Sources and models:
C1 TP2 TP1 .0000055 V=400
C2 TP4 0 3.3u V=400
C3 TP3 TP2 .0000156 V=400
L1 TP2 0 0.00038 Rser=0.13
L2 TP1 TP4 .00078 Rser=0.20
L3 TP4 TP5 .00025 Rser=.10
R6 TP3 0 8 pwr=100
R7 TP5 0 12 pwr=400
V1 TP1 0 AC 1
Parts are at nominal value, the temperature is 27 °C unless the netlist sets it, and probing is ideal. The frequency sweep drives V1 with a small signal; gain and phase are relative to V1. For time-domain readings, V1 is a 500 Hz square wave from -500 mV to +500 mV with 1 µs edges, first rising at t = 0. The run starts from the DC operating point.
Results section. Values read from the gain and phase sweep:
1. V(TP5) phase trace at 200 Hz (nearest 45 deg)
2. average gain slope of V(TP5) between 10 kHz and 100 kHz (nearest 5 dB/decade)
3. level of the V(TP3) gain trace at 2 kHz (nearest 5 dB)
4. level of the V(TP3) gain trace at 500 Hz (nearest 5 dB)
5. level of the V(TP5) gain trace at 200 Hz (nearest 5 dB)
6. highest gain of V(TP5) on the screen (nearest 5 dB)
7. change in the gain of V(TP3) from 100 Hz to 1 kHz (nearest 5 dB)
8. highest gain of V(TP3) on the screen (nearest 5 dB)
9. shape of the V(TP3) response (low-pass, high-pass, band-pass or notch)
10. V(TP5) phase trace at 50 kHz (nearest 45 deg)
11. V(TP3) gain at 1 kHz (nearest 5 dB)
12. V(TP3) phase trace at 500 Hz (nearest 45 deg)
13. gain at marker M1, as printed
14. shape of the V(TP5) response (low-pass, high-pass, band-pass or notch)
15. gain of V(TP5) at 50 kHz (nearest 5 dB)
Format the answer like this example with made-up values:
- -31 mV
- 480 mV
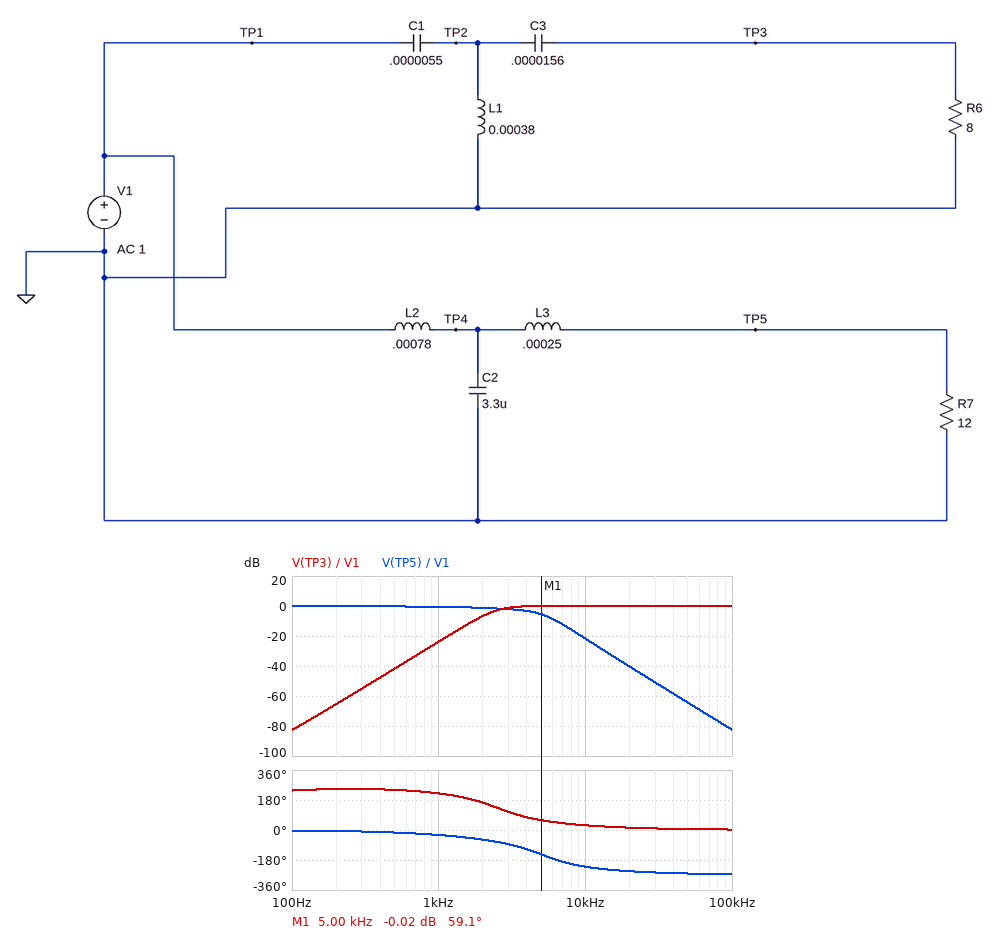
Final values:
- 0 deg
- -60 dB/decade
- -5 dB
- -40 dB
- 0 dB
- 0 dB
- 60 dB
- 0 dB
- high-pass
- -270 deg
- -25 dB
- 225 deg
- -0.02 dB
- low-pass
- -65 dB
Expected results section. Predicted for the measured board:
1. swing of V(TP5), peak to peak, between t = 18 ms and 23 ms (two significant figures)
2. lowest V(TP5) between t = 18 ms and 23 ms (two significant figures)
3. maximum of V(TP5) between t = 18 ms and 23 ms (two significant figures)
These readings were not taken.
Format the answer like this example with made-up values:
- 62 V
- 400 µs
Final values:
- 980 mV
- -490 mV
- 490 mV
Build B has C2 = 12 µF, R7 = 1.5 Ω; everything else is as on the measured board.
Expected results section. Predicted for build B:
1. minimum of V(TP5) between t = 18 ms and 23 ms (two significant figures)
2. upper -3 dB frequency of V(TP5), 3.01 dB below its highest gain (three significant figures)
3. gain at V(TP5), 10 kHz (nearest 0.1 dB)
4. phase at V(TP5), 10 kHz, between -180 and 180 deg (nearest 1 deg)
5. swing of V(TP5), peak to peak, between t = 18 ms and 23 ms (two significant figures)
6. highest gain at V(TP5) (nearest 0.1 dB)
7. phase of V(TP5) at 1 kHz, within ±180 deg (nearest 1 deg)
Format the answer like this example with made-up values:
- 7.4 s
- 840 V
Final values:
- -290 mV
- 287 Hz
- -50.8 dB
- 97 deg
- 590 mV
- -1.6 dB
- -79 deg
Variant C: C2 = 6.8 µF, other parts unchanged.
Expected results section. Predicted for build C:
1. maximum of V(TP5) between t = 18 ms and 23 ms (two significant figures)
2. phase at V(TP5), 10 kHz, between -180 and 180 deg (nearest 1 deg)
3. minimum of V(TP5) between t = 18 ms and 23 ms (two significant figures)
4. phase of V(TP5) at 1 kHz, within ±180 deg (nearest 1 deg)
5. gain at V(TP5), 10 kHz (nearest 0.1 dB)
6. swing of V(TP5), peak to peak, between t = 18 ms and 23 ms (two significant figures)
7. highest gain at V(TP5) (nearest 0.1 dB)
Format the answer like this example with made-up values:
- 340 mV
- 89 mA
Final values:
- 650 mV
- 133 deg
- -650 mV
- -33 deg
- -29.5 dB
- 1.3 V
- 1.0 dB
